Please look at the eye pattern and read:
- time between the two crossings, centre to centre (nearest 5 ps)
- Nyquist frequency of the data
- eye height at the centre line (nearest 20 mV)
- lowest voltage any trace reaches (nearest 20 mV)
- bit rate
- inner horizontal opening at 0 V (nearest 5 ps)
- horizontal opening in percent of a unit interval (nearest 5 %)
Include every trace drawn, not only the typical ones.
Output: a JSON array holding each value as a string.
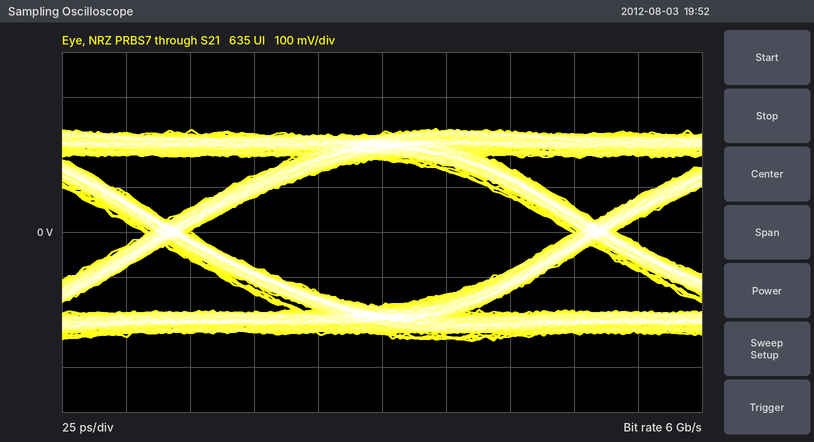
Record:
["165 ps", "3 GHz", "320 mV", "-240 mV", "6 Gb/s", "150 ps", "90 %"]
